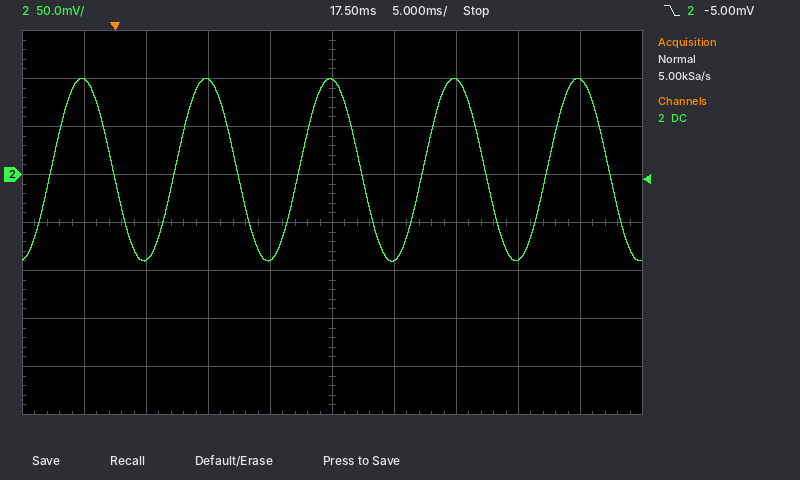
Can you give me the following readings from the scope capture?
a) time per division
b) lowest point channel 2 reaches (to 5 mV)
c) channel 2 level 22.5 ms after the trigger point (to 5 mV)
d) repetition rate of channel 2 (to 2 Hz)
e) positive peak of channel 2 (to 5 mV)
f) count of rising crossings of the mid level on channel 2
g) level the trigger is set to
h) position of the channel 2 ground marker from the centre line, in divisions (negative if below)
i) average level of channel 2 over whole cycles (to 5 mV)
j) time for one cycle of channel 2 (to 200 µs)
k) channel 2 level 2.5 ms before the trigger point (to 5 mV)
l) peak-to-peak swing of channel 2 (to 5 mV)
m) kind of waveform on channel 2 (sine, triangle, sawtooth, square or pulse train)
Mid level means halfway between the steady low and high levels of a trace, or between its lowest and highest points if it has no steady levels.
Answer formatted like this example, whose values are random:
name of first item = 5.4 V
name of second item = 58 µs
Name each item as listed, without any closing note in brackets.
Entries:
time per division = 5 ms
lowest point channel 2 reaches = -90 mV
channel 2 level 22.5 ms after the trigger point = -90 mV
repetition rate of channel 2 = 100 Hz
positive peak of channel 2 = 100 mV
count of rising crossings of the mid level on channel 2 = 5
level the trigger is set to = -5.00 mV
position of the channel 2 ground marker from the centre line, in divisions = +1.0 div
average level of channel 2 over whole cycles = 5 mV
time for one cycle of channel 2 = 10.0 ms
channel 2 level 2.5 ms before the trigger point = 100 mV
peak-to-peak swing of channel 2 = 190 mV
kind of waveform on channel 2 = sine
